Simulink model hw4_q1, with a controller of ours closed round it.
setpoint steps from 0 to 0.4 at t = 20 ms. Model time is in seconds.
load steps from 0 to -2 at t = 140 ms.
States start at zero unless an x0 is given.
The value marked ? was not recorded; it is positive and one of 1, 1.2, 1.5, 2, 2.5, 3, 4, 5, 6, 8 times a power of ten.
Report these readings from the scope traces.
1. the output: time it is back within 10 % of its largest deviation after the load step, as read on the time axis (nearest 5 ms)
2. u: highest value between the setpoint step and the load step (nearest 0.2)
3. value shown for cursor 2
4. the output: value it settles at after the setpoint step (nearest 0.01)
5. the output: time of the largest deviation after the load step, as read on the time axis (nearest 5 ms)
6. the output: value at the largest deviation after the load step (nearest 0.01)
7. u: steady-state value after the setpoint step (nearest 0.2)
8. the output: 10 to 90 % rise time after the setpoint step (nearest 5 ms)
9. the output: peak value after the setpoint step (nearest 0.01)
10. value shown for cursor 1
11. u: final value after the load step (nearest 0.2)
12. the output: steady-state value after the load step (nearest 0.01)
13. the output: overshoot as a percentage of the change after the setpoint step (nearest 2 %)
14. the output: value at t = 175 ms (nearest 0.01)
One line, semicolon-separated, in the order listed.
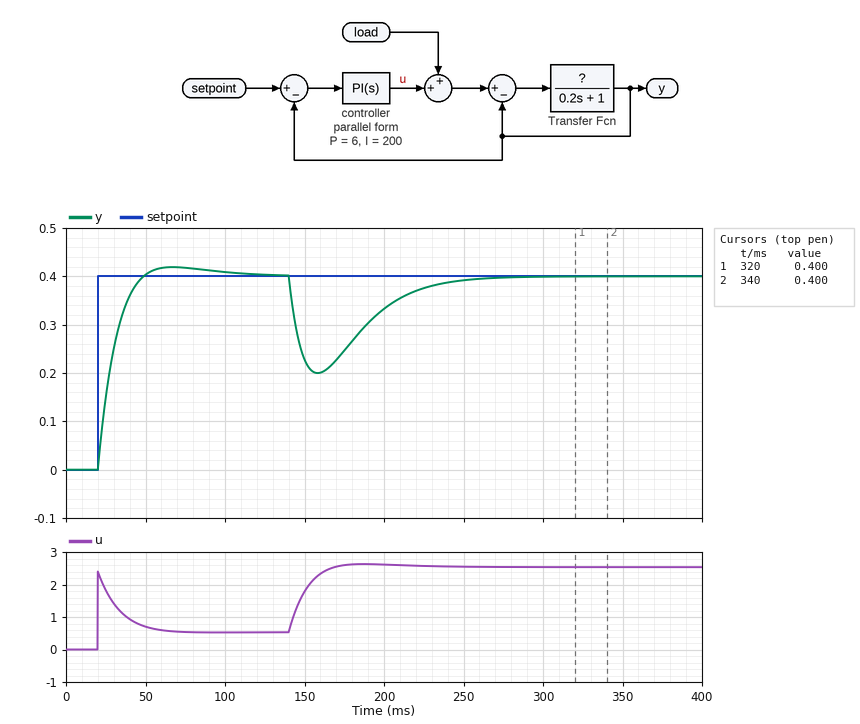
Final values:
230 ms; 2.4; 0.400; 0.40; 160 ms; 0.20; 0.6; 20 ms; 0.42; 0.400; 2.6; 0.40; 4 %; 0.25
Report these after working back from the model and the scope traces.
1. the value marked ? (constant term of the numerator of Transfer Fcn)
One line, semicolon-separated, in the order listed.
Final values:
3
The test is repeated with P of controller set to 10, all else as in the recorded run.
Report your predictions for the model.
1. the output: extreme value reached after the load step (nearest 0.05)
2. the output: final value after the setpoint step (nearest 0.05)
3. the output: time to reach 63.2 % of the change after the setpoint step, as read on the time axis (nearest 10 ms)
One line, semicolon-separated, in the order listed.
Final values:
0.25; 0.40; 30 ms
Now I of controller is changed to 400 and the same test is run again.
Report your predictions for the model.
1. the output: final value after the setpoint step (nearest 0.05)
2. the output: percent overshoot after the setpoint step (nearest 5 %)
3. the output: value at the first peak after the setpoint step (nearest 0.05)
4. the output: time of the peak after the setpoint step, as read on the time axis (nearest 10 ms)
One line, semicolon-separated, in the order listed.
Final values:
0.40; 15 %; 0.45; 50 ms
